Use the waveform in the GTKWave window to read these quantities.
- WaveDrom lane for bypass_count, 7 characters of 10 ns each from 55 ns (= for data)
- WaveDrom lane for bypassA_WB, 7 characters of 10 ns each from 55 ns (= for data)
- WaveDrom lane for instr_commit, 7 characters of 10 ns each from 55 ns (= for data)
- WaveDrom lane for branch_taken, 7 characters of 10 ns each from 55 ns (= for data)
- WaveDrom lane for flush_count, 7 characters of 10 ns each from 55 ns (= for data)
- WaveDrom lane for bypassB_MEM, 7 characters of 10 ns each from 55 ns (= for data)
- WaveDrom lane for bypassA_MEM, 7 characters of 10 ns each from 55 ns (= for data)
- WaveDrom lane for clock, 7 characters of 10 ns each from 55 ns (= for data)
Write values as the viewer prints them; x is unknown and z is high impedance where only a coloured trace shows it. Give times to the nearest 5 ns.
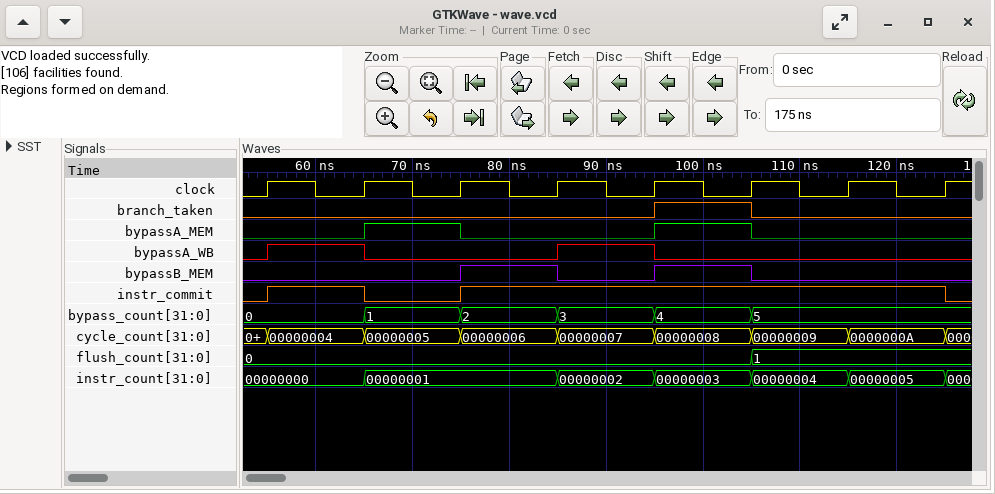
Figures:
{name: 'bypass_count', wave: '======.', data: '0 1 2 3 4 5'}
{name: 'bypassA_WB', wave: '10.10..'}
{name: 'instr_commit', wave: '101....'}
{name: 'branch_taken', wave: '0...10.'}
{name: 'flush_count', wave: '=....=.', data: '0 1'}
{name: 'bypassB_MEM', wave: '0.1010.'}
{name: 'bypassA_MEM', wave: '010.10.'}
{name: 'clock', wave: 'p......'}
